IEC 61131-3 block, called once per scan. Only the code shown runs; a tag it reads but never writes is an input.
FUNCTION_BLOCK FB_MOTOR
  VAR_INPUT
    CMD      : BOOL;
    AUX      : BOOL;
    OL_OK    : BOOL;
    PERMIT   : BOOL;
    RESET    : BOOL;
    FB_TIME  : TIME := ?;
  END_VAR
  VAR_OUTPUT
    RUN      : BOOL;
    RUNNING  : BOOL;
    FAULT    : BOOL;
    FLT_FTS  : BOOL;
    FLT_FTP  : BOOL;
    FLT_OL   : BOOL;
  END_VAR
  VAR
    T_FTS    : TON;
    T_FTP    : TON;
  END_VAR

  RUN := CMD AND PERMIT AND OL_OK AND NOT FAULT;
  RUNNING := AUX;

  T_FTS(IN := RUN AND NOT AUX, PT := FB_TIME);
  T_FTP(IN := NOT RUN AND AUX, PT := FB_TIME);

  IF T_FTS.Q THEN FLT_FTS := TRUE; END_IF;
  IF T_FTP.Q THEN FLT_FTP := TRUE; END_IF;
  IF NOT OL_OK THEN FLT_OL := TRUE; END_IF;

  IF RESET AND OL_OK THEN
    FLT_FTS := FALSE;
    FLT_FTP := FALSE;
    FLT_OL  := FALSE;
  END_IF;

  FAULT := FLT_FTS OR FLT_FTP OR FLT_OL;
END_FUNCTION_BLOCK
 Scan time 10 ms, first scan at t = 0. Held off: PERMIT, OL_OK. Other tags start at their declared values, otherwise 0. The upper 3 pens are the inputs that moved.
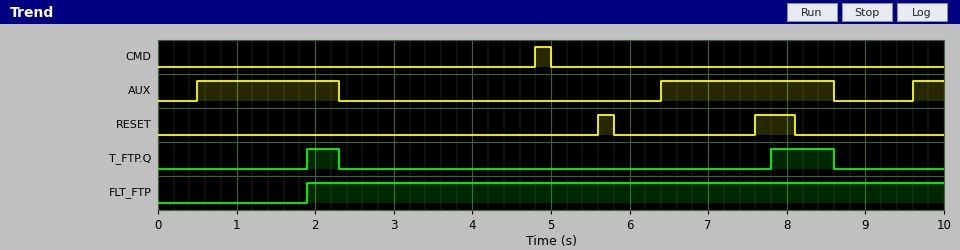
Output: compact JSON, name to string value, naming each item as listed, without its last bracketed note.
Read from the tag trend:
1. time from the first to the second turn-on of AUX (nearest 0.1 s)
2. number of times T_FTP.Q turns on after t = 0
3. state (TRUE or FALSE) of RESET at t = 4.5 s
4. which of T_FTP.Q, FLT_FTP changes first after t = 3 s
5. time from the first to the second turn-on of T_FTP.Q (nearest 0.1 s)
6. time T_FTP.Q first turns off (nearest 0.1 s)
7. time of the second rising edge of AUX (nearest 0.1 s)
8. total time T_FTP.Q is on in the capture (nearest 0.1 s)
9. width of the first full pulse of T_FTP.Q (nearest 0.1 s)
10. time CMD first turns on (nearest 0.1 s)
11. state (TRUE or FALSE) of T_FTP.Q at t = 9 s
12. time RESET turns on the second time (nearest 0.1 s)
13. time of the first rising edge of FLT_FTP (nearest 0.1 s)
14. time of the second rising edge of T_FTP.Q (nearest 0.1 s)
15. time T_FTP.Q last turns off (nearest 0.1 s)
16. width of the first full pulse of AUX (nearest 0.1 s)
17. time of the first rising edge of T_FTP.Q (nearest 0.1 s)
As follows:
{"time from the first to the second turn-on of AUX": "5.9 s", "number of times T_FTP.Q turns on after t = 0": "2", "state (TRUE or FALSE) of RESET at t = 4.5 s": "FALSE", "which of T_FTP.Q, FLT_FTP changes first after t = 3 s": "T_FTP.Q", "time from the first to the second turn-on of T_FTP.Q": "5.9 s", "time T_FTP.Q first turns off": "2.3 s", "time of the second rising edge of AUX": "6.4 s", "total time T_FTP.Q is on in the capture": "1.2 s", "width of the first full pulse of T_FTP.Q": "0.4 s", "time CMD first turns on": "4.8 s", "state (TRUE or FALSE) of T_FTP.Q at t = 9 s": "FALSE", "time RESET turns on the second time": "7.6 s", "time of the first rising edge of FLT_FTP": "1.9 s", "time of the second rising edge of T_FTP.Q": "7.8 s", "time T_FTP.Q last turns off": "8.6 s", "width of the first full pulse of AUX": "1.8 s", "time of the first rising edge of T_FTP.Q": "1.9 s"}
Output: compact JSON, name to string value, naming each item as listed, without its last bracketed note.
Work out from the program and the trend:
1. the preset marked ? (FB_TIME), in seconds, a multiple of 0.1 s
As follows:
{"the preset marked ? (FB_TIME), in seconds, a multiple of 0.1 s": "1.4 s"}
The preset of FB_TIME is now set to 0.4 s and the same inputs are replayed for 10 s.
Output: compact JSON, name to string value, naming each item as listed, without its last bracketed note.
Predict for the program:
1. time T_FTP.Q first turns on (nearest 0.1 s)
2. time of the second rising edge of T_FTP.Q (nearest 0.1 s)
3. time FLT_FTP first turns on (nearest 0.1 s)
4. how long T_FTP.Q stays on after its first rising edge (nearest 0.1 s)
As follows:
{"time T_FTP.Q first turns on": "0.9 s", "time of the second rising edge of T_FTP.Q": "6.8 s", "time FLT_FTP first turns on": "0.9 s", "how long T_FTP.Q stays on after its first rising edge": "1.4 s"}
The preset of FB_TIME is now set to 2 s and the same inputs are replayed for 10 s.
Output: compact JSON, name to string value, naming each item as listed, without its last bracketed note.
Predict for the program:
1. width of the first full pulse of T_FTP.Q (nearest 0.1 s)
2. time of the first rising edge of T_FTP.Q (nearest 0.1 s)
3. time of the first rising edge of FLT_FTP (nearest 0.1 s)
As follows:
{"width of the first full pulse of T_FTP.Q": "0.2 s", "time of the first rising edge of T_FTP.Q": "8.4 s", "time of the first rising edge of FLT_FTP": "8.4 s"}
